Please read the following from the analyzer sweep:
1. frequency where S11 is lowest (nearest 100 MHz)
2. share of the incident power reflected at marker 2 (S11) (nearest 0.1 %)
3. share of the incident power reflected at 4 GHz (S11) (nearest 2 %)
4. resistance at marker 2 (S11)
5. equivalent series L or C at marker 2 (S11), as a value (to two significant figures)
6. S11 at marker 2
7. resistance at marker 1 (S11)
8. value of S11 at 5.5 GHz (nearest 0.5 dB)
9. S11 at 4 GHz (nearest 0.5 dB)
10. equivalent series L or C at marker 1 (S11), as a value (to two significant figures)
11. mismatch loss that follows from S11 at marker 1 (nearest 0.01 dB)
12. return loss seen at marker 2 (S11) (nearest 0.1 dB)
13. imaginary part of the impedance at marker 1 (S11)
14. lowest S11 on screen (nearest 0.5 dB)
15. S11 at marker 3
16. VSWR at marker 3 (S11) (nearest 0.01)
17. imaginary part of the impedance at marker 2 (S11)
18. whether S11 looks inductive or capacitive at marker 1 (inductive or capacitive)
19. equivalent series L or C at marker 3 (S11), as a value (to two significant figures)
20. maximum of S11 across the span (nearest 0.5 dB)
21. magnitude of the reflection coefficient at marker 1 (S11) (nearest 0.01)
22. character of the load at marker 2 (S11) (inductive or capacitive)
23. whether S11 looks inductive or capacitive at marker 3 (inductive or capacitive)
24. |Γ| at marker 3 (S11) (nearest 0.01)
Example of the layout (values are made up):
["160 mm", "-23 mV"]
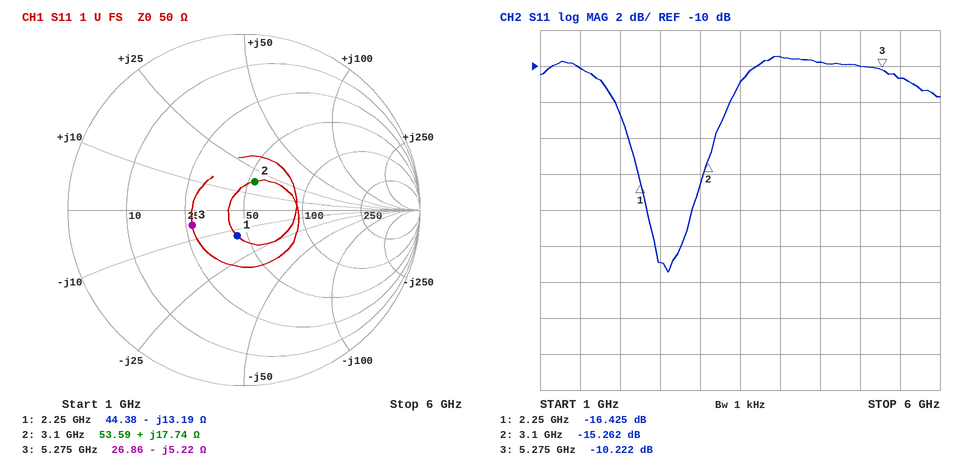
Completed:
["2.6 GHz", "3.0 %", "12 %", "53.59 Ω", "910 pH", "-15.262 dB", "44.38 Ω", "-10.5 dB", "-9.5 dB", "5.4 pF", "0.10 dB", "15.3 dB", "-13.19 Ω", "-21.5 dB", "-10.222 dB", "1.89", "+17.74 Ω", "capacitive", "5.8 pF", "-9.5 dB", "0.15", "inductive", "capacitive", "0.31"]
